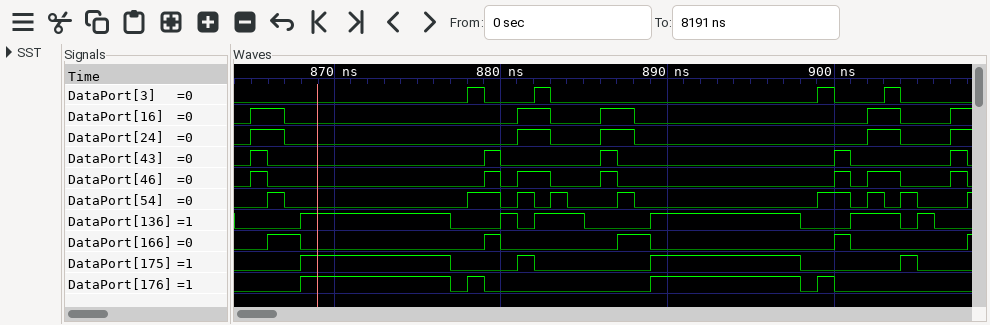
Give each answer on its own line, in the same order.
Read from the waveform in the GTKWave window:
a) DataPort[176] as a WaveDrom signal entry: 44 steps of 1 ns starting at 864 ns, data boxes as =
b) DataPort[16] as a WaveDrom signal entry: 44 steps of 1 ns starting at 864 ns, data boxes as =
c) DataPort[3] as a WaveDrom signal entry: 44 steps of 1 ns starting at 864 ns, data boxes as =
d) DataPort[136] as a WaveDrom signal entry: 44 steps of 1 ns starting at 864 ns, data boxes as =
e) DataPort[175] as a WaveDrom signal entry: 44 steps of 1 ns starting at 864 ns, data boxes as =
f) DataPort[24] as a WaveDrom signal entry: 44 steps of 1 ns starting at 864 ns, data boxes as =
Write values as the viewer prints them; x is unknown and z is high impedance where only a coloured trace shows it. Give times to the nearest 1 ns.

{name: 'DataPort[176]', wave: '0...1........010.........1........010.......'}
{name: 'DataPort[16]', wave: '01.0.............1.0..1.0.............1.0..1'}
{name: 'DataPort[3]', wave: '0.............10..10...............10..10...'}
{name: 'DataPort[136]', wave: '0...1........0..101..0...1........0..1..010.'}
{name: 'DataPort[175]', wave: '0...1........0...10......1........0.....10..'}
{name: 'DataPort[24]', wave: '01.0.............1.0..1.0.............1.0..1'}
